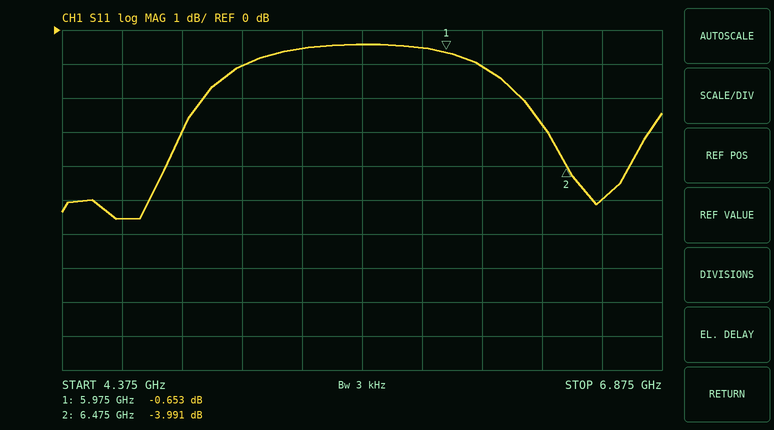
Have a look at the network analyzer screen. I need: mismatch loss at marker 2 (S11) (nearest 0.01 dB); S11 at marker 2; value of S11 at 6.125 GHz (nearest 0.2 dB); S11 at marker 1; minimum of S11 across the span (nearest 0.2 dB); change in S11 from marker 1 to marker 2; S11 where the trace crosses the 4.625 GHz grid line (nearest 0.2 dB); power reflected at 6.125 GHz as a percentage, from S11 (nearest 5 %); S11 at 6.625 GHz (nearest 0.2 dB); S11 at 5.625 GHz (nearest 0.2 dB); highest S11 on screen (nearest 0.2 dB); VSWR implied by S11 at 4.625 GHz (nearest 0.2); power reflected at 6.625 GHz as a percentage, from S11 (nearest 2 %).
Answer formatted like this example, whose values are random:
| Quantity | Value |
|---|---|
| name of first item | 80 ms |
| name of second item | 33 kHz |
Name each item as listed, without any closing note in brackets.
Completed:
| Quantity | Value |
|---|---|
| mismatch loss at marker 2 (S11) | 2.21 dB |
| S11 at marker 2 | -3.991 dB |
| value of S11 at 6.125 GHz | -1.0 dB |
| S11 at marker 1 | -0.653 dB |
| minimum of S11 across the span | -5.6 dB |
| change in S11 from marker 1 to marker 2 | -3.338 dB |
| S11 where the trace crosses the 4.625 GHz grid line | -5.6 dB |
| power reflected at 6.125 GHz as a percentage, from S11 | 80 % |
| S11 at 6.625 GHz | -5.0 dB |
| S11 at 5.625 GHz | -0.4 dB |
| highest S11 on screen | -0.4 dB |
| VSWR implied by S11 at 4.625 GHz | 3.2 |
| power reflected at 6.625 GHz as a percentage, from S11 | 32 % |
